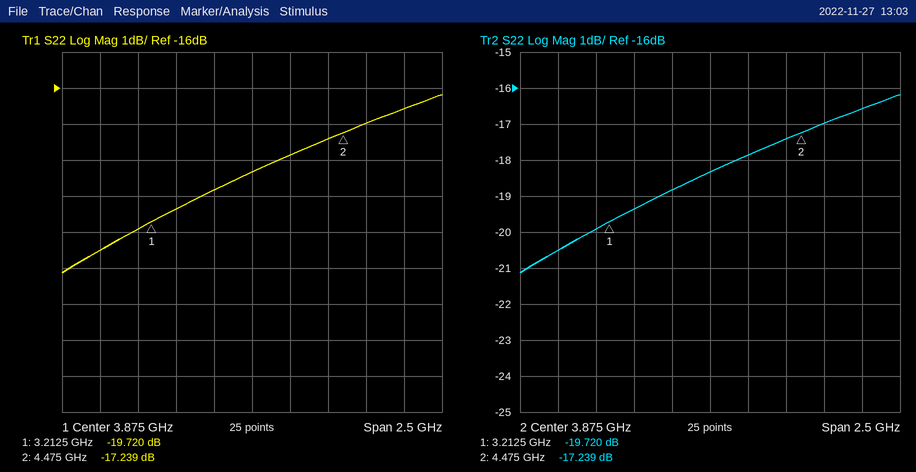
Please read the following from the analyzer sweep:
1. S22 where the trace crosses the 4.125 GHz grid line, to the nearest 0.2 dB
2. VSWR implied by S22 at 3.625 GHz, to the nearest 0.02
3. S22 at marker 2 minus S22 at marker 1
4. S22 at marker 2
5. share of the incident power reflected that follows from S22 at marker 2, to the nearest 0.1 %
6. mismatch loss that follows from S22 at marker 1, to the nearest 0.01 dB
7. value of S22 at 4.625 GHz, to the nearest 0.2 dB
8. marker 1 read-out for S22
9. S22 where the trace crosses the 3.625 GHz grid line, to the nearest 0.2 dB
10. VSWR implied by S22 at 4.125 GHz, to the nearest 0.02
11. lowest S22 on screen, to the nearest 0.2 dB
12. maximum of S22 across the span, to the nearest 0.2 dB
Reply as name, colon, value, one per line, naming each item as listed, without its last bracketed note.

S22 where the trace crosses the 4.125 GHz grid line, to the nearest 0.2 dB: -17.8 dB
VSWR implied by S22 at 3.625 GHz, to the nearest 0.02: 1.26
S22 at marker 2 minus S22 at marker 1: 2.481 dB
S22 at marker 2: -17.239 dB
share of the incident power reflected that follows from S22 at marker 2, to the nearest 0.1 %: 1.9 %
mismatch loss that follows from S22 at marker 1, to the nearest 0.01 dB: 0.05 dB
value of S22 at 4.625 GHz, to the nearest 0.2 dB: -17.0 dB
marker 1 read-out for S22: -19.720 dB
S22 where the trace crosses the 3.625 GHz grid line, to the nearest 0.2 dB: -18.8 dB
VSWR implied by S22 at 4.125 GHz, to the nearest 0.02: 1.30
lowest S22 on screen, to the nearest 0.2 dB: -21.2 dB
maximum of S22 across the span, to the nearest 0.2 dB: -16.2 dB
